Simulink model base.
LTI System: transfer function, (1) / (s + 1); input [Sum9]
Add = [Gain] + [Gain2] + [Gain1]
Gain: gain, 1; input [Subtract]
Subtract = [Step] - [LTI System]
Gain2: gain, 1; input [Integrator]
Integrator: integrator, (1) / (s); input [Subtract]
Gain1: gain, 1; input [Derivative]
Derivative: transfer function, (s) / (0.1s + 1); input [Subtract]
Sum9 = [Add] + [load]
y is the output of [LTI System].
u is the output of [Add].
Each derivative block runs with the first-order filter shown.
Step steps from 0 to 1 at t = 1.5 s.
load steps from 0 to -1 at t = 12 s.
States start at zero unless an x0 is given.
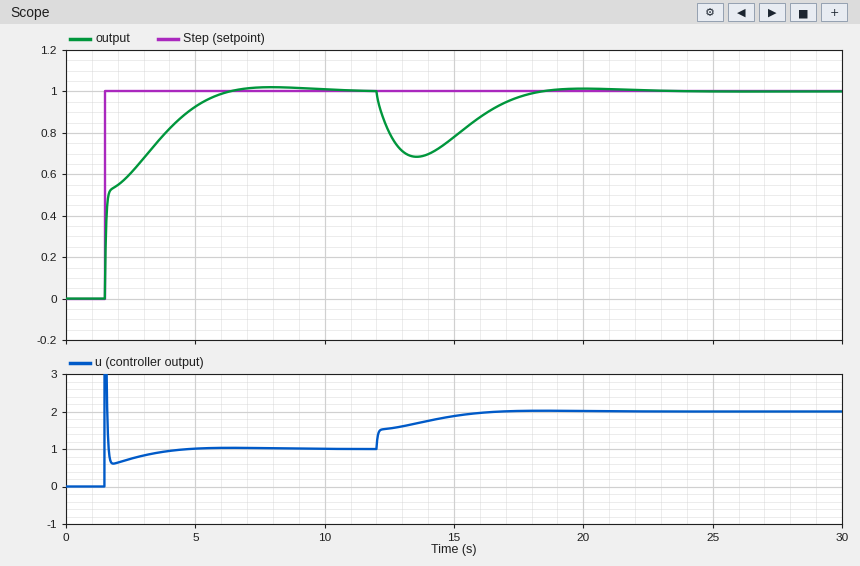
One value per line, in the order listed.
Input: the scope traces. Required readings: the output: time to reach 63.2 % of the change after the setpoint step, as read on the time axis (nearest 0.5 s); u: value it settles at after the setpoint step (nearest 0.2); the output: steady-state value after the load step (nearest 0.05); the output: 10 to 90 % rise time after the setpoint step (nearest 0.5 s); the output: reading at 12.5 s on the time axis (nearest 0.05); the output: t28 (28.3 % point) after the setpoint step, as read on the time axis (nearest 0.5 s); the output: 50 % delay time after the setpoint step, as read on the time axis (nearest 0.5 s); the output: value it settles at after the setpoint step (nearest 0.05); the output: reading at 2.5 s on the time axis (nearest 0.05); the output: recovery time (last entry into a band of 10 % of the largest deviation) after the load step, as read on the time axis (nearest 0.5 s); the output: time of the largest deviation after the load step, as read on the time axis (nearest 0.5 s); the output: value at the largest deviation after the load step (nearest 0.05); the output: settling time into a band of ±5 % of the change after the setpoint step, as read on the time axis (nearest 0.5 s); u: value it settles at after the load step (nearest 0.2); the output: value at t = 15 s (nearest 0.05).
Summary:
2.5 s
1.0
1.00
3.0 s
0.80
1.5 s
1.5 s
1.00
0.60
17.5 s
13.5 s
0.70
5.5 s
2.0
0.80
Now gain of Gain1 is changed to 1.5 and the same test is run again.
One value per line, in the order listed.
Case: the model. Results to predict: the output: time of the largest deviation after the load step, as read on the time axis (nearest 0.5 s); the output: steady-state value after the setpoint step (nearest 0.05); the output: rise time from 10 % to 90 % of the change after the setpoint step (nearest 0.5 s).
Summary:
14.0 s
1.00
3.5 s
